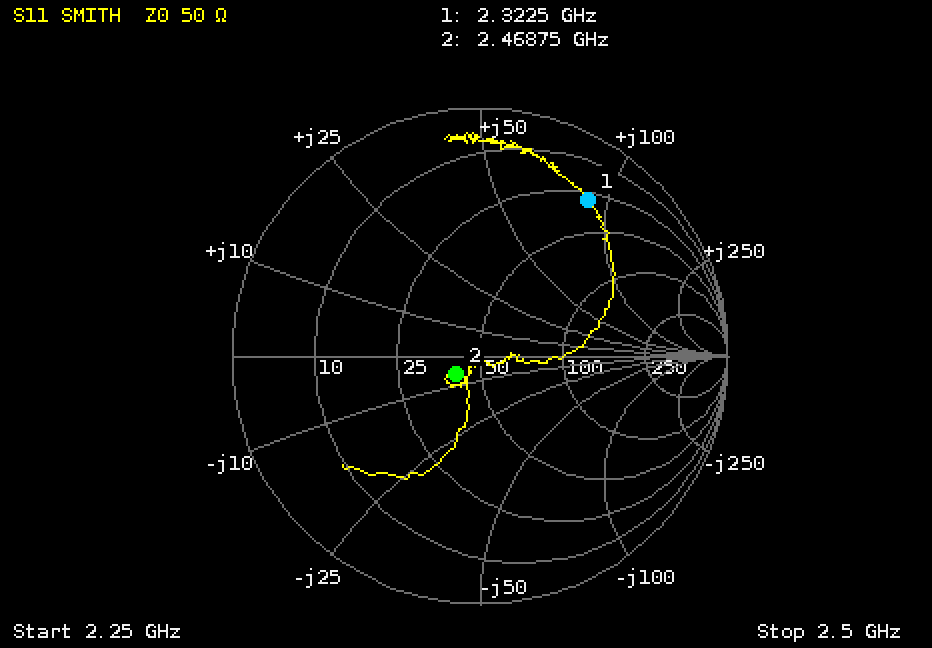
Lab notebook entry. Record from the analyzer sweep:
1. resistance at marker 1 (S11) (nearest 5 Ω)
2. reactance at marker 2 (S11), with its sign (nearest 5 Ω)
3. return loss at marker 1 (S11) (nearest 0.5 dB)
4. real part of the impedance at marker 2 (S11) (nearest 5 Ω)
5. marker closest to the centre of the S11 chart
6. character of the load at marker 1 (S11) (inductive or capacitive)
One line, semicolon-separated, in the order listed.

30 Ω; -5 Ω; 2.5 dB; 40 Ω; marker 2; inductive
